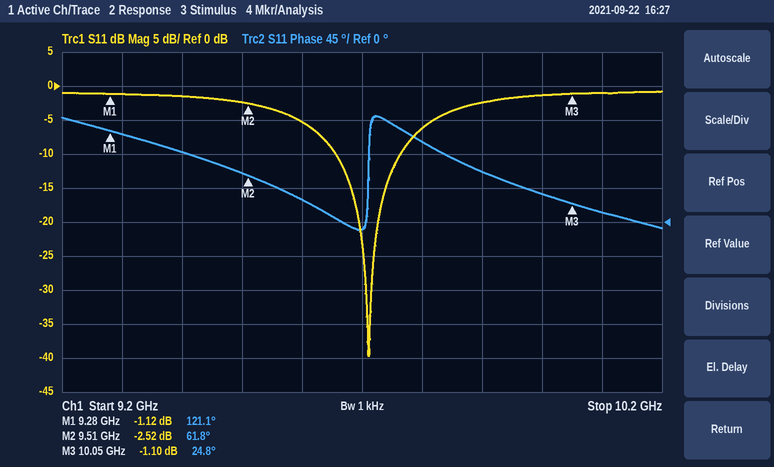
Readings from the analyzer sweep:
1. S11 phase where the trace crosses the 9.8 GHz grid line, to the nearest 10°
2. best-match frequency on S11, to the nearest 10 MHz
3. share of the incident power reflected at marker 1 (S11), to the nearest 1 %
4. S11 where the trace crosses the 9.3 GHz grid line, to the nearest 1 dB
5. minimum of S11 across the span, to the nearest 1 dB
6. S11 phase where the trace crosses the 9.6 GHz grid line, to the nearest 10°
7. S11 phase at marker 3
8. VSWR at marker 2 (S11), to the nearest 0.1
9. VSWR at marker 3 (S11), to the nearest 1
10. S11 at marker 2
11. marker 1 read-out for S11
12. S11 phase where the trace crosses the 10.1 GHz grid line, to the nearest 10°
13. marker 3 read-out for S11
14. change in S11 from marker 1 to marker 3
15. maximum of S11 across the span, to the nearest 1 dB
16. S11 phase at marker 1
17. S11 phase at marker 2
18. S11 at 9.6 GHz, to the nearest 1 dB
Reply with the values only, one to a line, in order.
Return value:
110°
9.71 GHz
77 %
-1 dB
-40 dB
30°
24.8°
6.9
16
-2.52 dB
-1.12 dB
10°
-1.10 dB
0.02 dB
-1 dB
121.1°
61.8°
-5 dB
